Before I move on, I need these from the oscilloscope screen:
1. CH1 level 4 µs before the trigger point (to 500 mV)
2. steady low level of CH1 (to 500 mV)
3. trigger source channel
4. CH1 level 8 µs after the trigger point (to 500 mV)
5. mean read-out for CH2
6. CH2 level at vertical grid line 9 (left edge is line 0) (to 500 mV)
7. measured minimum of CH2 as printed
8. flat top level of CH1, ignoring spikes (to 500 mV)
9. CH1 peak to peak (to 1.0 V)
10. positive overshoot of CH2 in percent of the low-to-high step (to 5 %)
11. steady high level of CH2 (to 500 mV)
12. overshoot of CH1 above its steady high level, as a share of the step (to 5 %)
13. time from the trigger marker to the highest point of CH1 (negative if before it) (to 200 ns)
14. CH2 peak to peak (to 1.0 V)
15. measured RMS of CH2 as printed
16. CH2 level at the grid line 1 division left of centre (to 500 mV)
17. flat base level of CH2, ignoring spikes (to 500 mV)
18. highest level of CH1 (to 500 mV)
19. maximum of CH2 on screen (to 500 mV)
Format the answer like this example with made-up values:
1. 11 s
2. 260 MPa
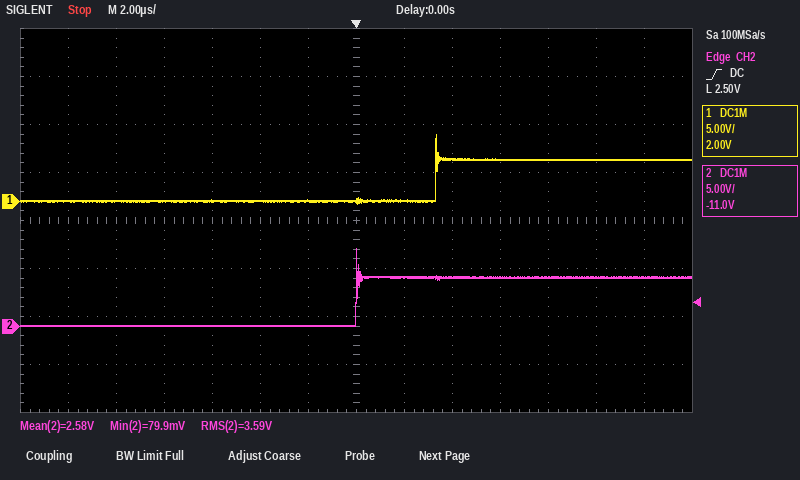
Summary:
1. 0.0 V
2. 0.0 V
3. CH2
4. 4.5 V
5. 2.58 V
6. 5.0 V
7. 79.9 mV
8. 4.5 V
9. 7.0 V
10. 60 %
11. 5.0 V
12. 60 %
13. +3.4 µs
14. 8.0 V
15. 3.59 V
16. 0.0 V
17. 0.0 V
18. 7.0 V
19. 8.0 V
